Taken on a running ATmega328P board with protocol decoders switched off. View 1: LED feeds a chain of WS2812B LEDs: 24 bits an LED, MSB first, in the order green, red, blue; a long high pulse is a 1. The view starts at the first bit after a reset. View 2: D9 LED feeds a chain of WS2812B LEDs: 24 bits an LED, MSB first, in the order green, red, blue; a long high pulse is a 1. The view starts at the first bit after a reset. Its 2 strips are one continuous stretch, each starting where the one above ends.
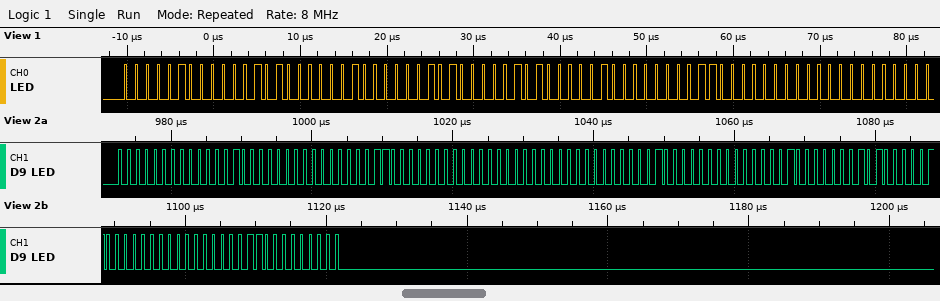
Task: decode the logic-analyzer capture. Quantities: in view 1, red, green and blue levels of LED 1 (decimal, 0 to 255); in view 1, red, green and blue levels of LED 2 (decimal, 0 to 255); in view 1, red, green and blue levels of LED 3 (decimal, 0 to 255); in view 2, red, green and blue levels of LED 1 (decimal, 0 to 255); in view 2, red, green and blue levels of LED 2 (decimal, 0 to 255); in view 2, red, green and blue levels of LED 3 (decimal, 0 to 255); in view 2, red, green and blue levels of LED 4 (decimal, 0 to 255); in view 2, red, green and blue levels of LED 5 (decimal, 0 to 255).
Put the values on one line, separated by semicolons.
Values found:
10, 4, 4; 10, 10, 8; 0, 6, 0; 4, 0, 0; 0, 6, 0; 4, 0, 0; 10, 8, 8; 6, 0, 0
